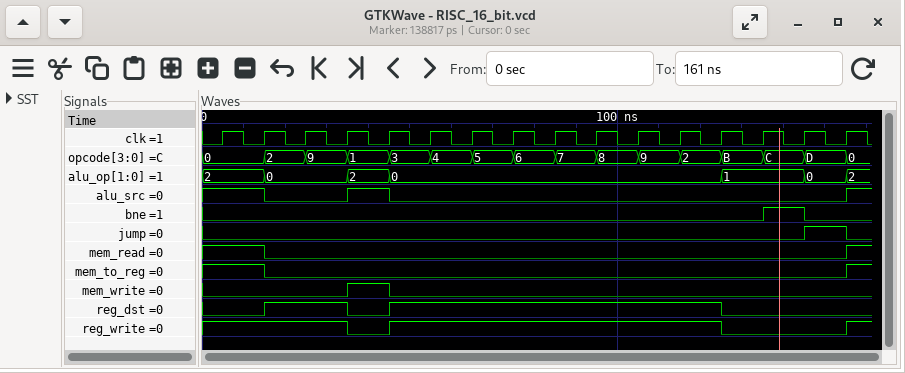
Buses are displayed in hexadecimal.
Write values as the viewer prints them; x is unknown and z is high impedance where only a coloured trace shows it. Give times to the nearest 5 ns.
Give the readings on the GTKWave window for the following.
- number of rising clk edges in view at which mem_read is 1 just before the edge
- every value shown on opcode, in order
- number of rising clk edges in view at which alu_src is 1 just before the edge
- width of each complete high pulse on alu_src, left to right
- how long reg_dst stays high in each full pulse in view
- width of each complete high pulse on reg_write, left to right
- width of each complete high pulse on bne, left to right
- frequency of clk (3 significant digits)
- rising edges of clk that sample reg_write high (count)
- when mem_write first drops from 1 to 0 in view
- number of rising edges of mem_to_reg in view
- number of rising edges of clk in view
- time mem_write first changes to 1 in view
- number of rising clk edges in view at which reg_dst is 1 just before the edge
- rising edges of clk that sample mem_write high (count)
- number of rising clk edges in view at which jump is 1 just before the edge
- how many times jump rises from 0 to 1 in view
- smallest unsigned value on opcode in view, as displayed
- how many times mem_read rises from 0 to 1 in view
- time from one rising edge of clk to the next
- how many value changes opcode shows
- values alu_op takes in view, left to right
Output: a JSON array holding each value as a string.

["2", "0, 2, 9, 1, 3, 4, 5, 6, 7, 8, 9, 2, B, C, D, 0", "3", "10 ns", "20 ns, 80 ns", "80 ns", "10 ns", "100 MHz", "12", "45 ns", "1", "16", "35 ns", "10", "1", "1", "1", "0", "1", "10 ns", "15", "2, 0, 2, 0, 1, 0, 2"]
